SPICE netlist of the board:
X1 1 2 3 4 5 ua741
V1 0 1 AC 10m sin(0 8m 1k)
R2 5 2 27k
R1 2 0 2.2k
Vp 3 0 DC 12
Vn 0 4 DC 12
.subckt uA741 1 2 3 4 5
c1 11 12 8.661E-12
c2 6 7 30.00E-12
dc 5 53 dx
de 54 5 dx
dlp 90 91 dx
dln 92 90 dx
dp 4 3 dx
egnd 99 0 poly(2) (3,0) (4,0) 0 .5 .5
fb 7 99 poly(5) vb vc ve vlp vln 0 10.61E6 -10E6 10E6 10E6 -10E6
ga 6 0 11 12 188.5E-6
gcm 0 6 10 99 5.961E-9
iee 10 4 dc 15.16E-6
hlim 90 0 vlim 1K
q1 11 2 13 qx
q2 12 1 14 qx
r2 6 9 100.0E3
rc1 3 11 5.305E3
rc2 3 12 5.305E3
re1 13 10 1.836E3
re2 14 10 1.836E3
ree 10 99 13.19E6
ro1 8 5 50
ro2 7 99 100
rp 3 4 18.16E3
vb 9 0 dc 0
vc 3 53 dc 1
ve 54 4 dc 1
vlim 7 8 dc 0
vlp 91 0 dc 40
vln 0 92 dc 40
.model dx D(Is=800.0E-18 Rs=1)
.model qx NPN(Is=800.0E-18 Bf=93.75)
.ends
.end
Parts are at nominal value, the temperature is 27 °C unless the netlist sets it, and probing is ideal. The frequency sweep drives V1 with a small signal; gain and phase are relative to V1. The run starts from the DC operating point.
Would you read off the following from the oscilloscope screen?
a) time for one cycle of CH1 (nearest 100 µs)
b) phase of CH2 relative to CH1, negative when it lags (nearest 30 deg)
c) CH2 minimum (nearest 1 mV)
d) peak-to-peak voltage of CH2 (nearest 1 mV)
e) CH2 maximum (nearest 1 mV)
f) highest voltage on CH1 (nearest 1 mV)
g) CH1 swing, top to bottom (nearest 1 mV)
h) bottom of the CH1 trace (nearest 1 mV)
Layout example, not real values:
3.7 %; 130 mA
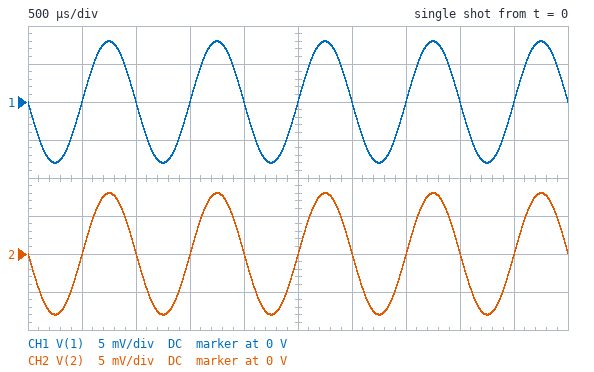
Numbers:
1.0 ms; 0 deg; -8 mV; 16 mV; 8 mV; 8 mV; 16 mV; -8 mV
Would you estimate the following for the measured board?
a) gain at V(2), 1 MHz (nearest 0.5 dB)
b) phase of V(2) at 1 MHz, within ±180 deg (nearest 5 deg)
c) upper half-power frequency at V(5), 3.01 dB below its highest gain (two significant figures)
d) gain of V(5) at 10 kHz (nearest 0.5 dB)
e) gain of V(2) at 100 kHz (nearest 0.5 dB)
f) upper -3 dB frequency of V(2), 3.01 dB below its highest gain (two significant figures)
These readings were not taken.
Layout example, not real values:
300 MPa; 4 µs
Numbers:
-23.5 dB; 65 deg; 78 kHz; 22.5 dB; -4.0 dB; 78 kHz
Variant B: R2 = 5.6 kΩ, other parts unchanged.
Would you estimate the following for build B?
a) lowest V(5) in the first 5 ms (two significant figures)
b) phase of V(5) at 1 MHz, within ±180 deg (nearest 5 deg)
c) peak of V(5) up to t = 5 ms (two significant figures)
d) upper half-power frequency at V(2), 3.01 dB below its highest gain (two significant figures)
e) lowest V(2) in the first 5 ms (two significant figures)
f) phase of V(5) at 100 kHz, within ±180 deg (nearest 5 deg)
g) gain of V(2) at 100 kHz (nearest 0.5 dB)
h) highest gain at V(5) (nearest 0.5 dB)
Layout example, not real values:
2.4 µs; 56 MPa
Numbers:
-28 mV; 75 deg; 29 mV; 330 kHz; -8.0 mV; 160 deg; -0.5 dB; 11.0 dB
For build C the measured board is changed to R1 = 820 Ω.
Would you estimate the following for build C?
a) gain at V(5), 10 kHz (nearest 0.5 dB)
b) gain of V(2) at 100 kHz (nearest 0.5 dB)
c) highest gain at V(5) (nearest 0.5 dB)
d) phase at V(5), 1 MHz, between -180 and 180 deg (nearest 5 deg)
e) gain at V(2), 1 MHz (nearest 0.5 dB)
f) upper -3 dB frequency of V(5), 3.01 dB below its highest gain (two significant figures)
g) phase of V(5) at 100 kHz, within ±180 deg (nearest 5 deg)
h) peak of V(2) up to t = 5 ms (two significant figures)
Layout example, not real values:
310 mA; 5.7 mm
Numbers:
30.0 dB; -11.0 dB; 30.5 dB; 60 deg; -32.0 dB; 30 kHz; 105 deg; 8.0 mV
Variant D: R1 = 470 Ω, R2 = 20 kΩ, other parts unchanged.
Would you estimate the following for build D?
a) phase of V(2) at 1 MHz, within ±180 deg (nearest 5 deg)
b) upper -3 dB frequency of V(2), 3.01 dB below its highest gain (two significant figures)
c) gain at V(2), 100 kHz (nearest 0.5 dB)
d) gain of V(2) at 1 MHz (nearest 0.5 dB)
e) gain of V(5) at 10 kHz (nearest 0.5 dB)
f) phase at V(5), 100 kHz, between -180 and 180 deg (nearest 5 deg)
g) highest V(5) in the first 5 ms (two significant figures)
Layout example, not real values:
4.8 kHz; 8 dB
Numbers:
60 deg; 23 kHz; -13.0 dB; -34.0 dB; 32.0 dB; 100 deg; 350 mV
